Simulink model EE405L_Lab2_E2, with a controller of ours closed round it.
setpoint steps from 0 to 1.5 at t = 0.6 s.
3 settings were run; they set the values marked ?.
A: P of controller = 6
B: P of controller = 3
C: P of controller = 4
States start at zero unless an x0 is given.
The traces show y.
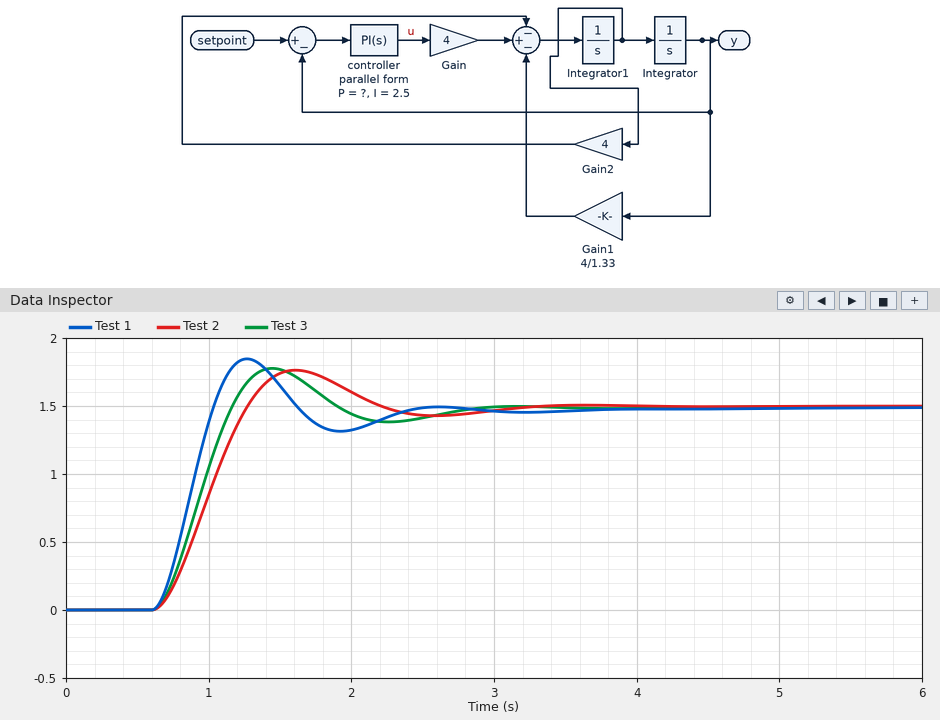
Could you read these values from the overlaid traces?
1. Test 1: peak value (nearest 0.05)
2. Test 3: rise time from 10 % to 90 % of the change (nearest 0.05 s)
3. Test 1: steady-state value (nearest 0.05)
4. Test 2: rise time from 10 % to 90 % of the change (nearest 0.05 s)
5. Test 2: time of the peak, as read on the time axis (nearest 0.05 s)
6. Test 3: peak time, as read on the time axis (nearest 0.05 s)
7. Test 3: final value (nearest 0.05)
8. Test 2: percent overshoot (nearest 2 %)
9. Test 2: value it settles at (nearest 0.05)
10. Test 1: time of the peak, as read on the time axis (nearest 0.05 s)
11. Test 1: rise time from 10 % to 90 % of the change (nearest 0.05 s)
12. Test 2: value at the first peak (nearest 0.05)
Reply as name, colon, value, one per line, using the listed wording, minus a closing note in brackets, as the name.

Test 1: peak value: 1.85
Test 3: rise time from 10 % to 90 % of the change: 0.40 s
Test 1: steady-state value: 1.50
Test 2: rise time from 10 % to 90 % of the change: 0.45 s
Test 2: time of the peak, as read on the time axis: 1.60 s
Test 3: peak time, as read on the time axis: 1.45 s
Test 3: final value: 1.50
Test 2: percent overshoot: 18 %
Test 2: value it settles at: 1.50
Test 1: time of the peak, as read on the time axis: 1.25 s
Test 1: rise time from 10 % to 90 % of the change: 0.30 s
Test 2: value at the first peak: 1.75
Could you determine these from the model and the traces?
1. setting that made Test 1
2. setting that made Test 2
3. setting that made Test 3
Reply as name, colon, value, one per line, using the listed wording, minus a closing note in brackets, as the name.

setting that made Test 1: A
setting that made Test 2: B
setting that made Test 3: C
